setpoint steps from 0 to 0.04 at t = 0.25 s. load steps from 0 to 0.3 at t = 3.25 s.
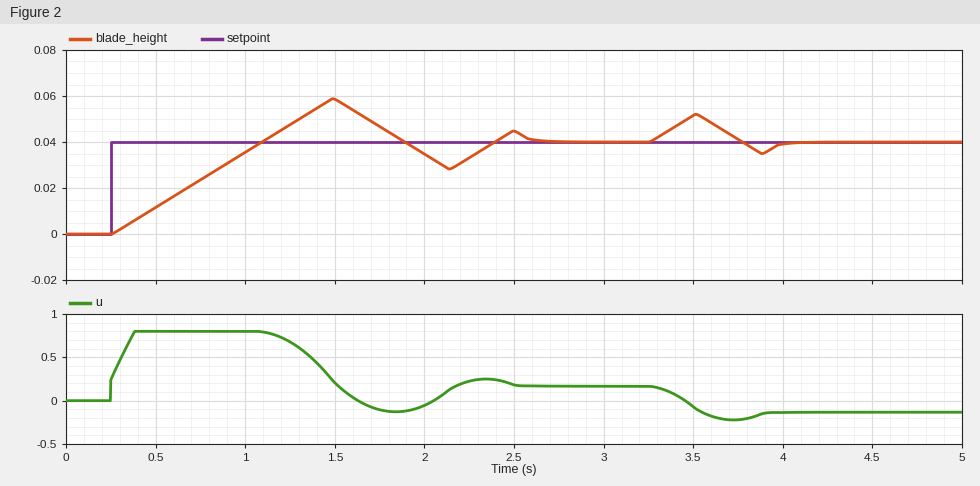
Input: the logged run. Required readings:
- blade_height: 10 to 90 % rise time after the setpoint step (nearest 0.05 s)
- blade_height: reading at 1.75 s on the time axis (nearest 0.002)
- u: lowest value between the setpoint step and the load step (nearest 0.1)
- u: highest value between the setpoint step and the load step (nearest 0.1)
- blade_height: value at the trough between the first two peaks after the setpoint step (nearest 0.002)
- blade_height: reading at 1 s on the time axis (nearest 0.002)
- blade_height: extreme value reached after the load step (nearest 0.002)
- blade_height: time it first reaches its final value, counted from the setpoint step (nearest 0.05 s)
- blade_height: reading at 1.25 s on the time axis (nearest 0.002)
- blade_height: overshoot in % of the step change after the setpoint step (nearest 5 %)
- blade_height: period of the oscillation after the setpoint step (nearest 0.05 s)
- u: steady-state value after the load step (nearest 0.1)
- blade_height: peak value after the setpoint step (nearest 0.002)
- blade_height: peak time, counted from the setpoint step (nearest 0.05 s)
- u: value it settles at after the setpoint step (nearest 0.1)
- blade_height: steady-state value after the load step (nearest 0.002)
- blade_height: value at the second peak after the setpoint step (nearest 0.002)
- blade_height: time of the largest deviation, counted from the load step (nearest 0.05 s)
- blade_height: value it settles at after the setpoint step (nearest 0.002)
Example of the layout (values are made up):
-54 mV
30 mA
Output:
0.65 s
0.046
-0.1
0.8
0.028
0.036
0.052
0.85 s
0.048
45 %
1.00 s
-0.1
0.058
1.25 s
0.2
0.040
0.044
0.25 s
0.040
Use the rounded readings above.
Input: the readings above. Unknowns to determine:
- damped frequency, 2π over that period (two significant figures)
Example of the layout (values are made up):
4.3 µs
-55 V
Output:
6.3 rad/s
